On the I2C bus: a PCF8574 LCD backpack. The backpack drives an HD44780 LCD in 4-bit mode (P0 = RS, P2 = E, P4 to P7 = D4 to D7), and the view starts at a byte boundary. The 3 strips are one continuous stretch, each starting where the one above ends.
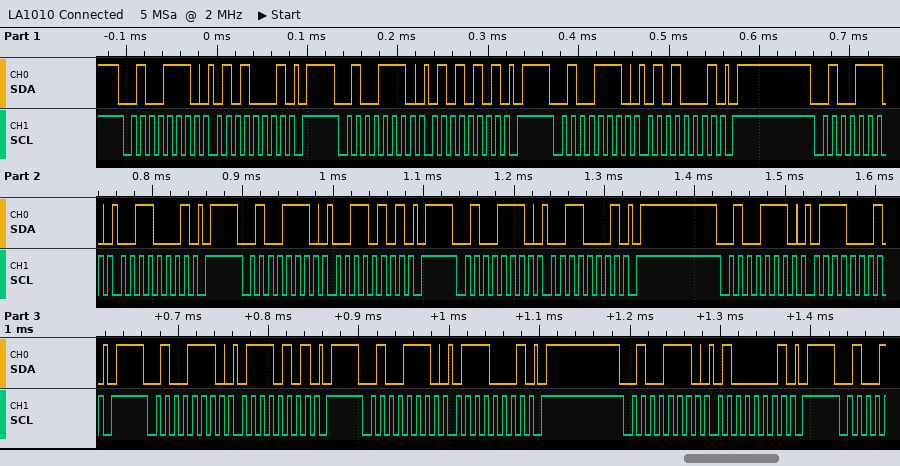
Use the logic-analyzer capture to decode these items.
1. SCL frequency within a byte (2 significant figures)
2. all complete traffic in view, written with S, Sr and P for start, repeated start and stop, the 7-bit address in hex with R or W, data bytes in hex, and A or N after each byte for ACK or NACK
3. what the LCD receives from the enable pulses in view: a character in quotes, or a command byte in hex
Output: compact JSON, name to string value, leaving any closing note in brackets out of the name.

{"SCL frequency within a byte": "100 kHz", "all complete traffic in view, written with S, Sr and P for start, repeated start and stop, the 7-bit address in hex with R or W, data bytes in hex, and A or N after each byte for ACK or NACK": "S 27W A 51 A P S 27W A 55 A P S 27W A 51 A P S 27W A 31 A P S 27W A 35 A P S 27W A 31 A P S 27W A 71 A P S 27W A 75 A P S 27W A 71 A P S 27W A 41 A P", "what the LCD receives from the enable pulses in view: a character in quotes, or a command byte in hex": "'S'"}
